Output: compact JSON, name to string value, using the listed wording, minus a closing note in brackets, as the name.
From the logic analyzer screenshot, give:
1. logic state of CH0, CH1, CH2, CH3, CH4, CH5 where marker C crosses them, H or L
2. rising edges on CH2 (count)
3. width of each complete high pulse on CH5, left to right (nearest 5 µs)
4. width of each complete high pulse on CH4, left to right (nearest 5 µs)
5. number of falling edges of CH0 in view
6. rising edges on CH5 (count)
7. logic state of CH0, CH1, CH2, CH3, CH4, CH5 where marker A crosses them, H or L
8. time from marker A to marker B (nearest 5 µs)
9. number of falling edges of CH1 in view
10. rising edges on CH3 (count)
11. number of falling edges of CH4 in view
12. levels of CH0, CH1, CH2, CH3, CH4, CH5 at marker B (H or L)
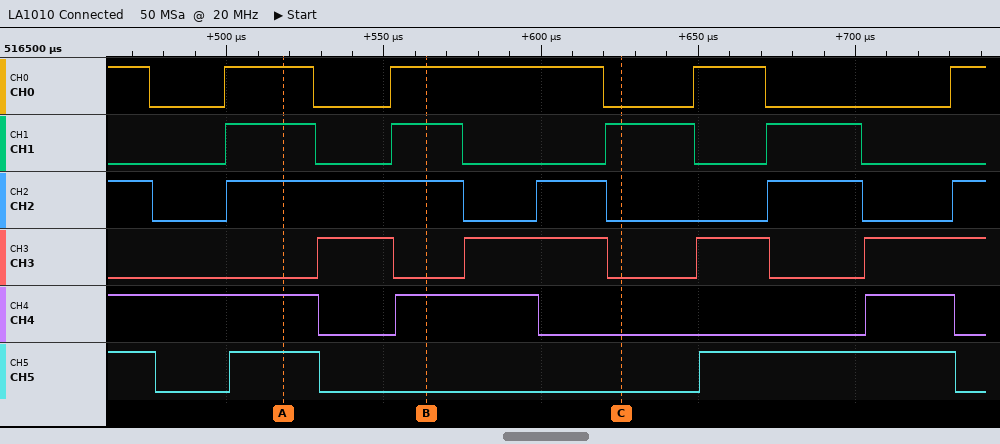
{"logic state of CH0, CH1, CH2, CH3, CH4, CH5 where marker C crosses them, H or L": "CH0=L, CH1=H, CH2=L, CH3=L, CH4=L, CH5=L", "rising edges on CH2": "4", "width of each complete high pulse on CH5, left to right": "30 µs, 80 µs", "width of each complete high pulse on CH4, left to right": "45 µs, 30 µs", "number of falling edges of CH0 in view": "4", "rising edges on CH5": "2", "logic state of CH0, CH1, CH2, CH3, CH4, CH5 where marker A crosses them, H or L": "CH0=H, CH1=H, CH2=H, CH3=L, CH4=H, CH5=H", "time from marker A to marker B": "45 µs", "number of falling edges of CH1 in view": "4", "rising edges on CH3": "4", "number of falling edges of CH4 in view": "3", "levels of CH0, CH1, CH2, CH3, CH4, CH5 at marker B": "CH0=H, CH1=H, CH2=H, CH3=L, CH4=H, CH5=L"}
